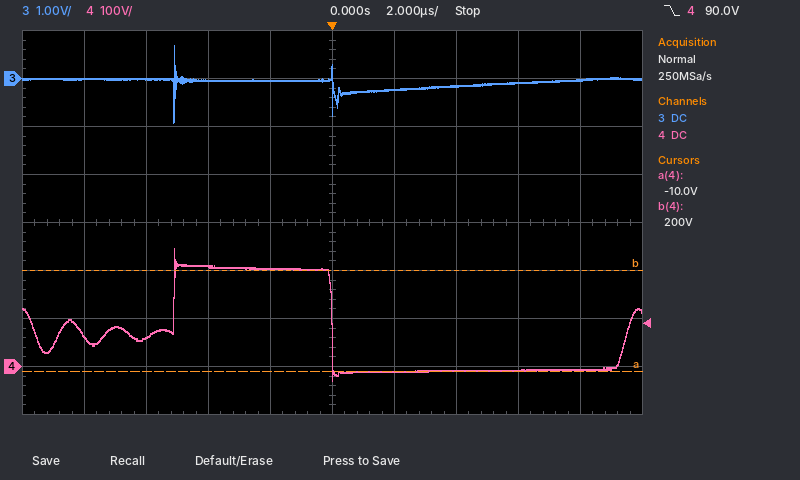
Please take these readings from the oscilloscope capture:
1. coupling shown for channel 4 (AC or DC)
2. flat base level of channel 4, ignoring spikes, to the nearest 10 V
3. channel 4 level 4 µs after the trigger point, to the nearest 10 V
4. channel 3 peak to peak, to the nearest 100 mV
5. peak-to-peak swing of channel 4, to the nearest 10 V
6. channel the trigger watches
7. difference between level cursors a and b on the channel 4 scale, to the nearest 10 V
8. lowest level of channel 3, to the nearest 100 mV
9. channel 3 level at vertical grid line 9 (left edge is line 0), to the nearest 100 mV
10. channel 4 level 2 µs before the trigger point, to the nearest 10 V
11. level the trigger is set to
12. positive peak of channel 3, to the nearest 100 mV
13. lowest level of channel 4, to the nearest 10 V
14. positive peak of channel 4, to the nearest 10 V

DC
-10 V
-10 V
1.6 V
280 V
channel 4
210 V
-900 mV
0.0 V
200 V
90.0 V
700 mV
-30 V
250 V
